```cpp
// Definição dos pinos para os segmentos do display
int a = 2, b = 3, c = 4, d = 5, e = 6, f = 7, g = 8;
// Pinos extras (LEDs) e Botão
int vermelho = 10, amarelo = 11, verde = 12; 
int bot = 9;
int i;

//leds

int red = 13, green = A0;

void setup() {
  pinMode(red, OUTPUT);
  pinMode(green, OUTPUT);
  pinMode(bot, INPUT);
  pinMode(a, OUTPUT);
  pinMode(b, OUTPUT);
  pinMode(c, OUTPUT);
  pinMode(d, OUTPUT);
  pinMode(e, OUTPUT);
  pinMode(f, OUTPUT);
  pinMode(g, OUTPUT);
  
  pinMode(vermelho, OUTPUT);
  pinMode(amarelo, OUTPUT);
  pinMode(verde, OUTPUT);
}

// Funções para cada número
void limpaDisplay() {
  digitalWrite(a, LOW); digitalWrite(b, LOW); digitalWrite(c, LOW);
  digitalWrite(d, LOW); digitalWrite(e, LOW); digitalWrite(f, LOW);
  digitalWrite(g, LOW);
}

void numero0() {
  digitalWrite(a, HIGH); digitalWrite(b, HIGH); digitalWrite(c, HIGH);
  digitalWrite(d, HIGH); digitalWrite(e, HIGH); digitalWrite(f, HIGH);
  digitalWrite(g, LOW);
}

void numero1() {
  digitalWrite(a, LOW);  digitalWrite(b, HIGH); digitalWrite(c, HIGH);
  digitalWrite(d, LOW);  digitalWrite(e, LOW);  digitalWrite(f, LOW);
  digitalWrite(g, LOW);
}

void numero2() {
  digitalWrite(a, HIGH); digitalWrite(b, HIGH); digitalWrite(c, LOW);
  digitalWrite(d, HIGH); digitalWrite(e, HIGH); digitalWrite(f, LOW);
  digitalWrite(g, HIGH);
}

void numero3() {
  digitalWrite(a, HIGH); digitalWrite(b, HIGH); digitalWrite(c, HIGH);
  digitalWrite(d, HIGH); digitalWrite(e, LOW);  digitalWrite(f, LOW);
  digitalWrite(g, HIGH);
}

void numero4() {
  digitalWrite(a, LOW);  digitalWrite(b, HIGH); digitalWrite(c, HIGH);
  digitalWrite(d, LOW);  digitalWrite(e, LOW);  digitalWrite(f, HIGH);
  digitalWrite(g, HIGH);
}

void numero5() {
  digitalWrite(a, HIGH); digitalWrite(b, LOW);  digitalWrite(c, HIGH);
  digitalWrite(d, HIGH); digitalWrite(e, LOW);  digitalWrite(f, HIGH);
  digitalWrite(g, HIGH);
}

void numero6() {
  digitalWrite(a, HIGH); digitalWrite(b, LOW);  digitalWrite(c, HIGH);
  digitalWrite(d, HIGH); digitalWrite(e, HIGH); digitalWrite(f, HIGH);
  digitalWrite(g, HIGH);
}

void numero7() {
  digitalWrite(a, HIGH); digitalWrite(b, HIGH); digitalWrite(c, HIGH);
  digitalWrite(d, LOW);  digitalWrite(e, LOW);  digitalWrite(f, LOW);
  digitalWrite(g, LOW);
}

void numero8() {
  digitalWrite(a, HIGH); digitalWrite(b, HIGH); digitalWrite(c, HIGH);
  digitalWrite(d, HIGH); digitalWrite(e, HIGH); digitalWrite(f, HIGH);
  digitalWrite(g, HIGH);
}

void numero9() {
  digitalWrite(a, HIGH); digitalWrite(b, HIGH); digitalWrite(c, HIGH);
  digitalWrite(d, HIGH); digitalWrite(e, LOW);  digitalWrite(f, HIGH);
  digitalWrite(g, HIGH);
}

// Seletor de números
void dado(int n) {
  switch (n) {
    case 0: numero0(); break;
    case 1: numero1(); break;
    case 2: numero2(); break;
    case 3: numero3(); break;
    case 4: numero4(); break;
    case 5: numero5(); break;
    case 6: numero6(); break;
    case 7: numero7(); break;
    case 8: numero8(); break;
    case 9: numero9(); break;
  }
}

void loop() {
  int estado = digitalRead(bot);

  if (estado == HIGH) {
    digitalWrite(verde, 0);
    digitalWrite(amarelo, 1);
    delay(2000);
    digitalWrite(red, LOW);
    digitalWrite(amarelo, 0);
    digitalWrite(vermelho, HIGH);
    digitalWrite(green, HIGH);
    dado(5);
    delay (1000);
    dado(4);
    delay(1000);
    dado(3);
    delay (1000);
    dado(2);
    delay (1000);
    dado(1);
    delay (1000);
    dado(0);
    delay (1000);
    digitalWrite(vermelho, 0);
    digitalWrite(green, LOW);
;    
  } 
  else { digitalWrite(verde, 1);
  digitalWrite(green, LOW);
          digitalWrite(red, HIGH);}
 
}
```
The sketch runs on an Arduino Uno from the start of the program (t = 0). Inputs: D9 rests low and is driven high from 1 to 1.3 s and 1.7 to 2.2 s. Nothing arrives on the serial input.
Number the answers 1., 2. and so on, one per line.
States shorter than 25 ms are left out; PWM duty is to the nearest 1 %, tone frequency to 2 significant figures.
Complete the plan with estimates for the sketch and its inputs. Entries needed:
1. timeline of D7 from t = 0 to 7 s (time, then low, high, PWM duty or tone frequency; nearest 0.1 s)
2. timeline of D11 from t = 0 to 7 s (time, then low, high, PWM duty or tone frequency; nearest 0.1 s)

1. 0 s low; 3 s high; 5 s low
2. 0 s low; 1 s high; 3 s low
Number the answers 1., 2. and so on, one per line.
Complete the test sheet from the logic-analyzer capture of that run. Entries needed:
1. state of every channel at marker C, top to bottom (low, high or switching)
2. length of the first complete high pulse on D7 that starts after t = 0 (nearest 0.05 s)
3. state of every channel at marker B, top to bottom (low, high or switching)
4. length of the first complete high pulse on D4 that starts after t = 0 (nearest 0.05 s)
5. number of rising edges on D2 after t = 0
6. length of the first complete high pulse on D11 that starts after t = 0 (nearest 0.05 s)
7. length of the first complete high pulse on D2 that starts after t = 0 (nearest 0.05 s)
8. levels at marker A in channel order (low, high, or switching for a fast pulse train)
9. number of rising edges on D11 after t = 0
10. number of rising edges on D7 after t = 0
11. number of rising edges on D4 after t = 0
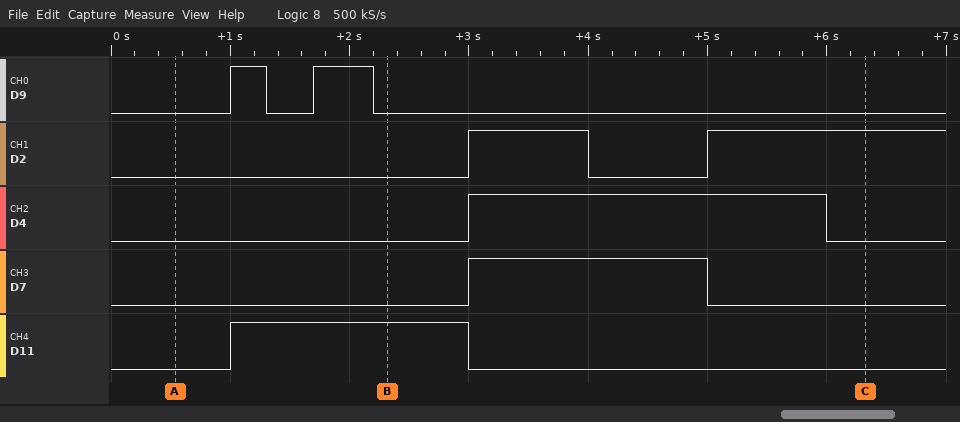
1. D9 low, D2 high, D4 low, D7 low, D11 low
2. 2.00 s
3. D9 low, D2 low, D4 low, D7 low, D11 high
4. 3.00 s
5. 2
6. 2.00 s
7. 1.00 s
8. D9 low, D2 low, D4 low, D7 low, D11 low
9. 1
10. 1
11. 1
